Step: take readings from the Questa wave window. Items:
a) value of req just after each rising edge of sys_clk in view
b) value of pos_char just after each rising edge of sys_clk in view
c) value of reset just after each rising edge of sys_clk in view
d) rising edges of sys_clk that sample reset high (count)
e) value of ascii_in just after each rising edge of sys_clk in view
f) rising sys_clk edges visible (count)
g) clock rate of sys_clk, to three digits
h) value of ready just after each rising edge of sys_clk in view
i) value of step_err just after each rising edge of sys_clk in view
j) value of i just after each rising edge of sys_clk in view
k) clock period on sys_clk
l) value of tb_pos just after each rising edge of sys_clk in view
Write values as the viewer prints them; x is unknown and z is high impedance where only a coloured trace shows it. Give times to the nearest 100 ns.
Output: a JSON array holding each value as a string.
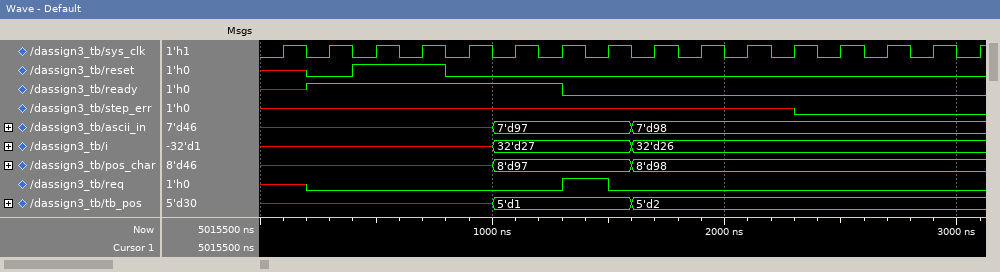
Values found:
["x 0 0 0 0 0 1 0 0 0 0 0 0 0 0 0", "x, x, x, x, x, 8'd97, 8'd97, 8'd97, 8'd98, 8'd98, 8'd98, 8'd98, 8'd98, 8'd98, 8'd98, 8'd98", "x 0 1 1 0 0 0 0 0 0 0 0 0 0 0 0", "2", "x, x, x, x, x, 7'd97, 7'd97, 7'd97, 7'd98, 7'd98, 7'd98, 7'd98, 7'd98, 7'd98, 7'd98, 7'd98", "16", "5.00 MHz", "x 1 1 1 1 1 0 0 0 0 0 0 0 0 0 0", "x x x x x x x x x x x 0 0 0 0 0", "x, x, x, x, x, 32'd27, 32'd27, 32'd27, 32'd26, 32'd26, 32'd26, 32'd26, 32'd26, 32'd26, 32'd26, 32'd26", "200 ns", "x, x, x, x, x, 5'd1, 5'd1, 5'd1, 5'd2, 5'd2, 5'd2, 5'd2, 5'd2, 5'd2, 5'd2, 5'd2"]
